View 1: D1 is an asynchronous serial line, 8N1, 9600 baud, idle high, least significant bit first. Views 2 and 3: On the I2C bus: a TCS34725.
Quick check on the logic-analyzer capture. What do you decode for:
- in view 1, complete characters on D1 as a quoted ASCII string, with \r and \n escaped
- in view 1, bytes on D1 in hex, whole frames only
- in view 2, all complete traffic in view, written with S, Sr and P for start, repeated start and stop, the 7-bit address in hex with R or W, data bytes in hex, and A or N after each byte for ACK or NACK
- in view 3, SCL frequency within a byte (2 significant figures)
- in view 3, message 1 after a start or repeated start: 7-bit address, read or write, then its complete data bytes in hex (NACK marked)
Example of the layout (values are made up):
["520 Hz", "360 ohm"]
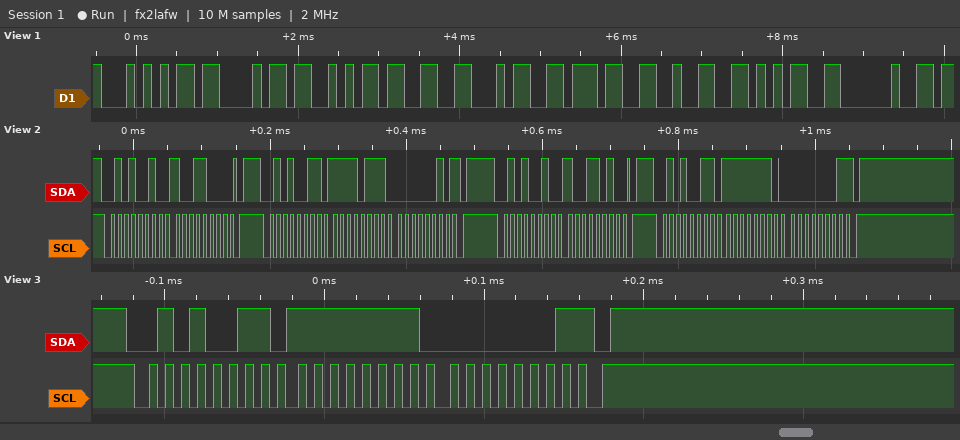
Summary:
["\"TCS34725 \"", "0x54 0x43 0x53 0x33 0x34 0x37 0x32 0x35 0x20", "S 29W A 98 A P S 29R A F7 A 02 N P S 29W A 9A A P S 29R A FE A 01 N P", "100 kHz", "0x29 read: FF 01 NACK"]
